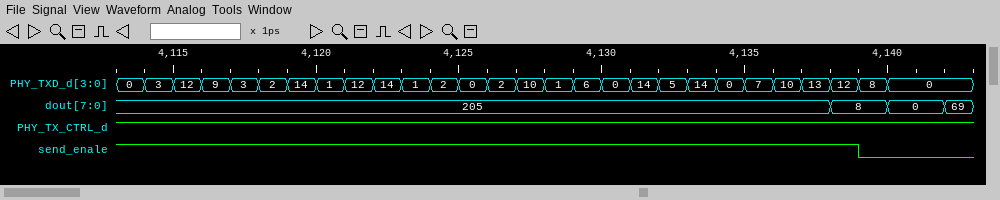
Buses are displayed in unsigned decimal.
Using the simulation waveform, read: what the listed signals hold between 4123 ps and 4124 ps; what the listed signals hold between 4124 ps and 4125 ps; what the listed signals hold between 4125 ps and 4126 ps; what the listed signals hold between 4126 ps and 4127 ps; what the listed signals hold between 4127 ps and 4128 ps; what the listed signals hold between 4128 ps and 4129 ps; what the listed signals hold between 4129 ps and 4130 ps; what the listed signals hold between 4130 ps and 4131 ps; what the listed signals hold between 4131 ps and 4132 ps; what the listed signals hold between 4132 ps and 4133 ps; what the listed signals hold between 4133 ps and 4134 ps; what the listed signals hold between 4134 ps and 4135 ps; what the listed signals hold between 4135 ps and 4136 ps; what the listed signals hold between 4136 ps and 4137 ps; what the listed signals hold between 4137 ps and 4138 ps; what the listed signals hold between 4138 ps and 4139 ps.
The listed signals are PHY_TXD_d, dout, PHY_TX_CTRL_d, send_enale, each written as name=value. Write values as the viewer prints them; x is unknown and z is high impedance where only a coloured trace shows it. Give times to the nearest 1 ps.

PHY_TXD_d=1, dout=205, PHY_TX_CTRL_d=1, send_enale=1
PHY_TXD_d=2, dout=205, PHY_TX_CTRL_d=1, send_enale=1
PHY_TXD_d=0, dout=205, PHY_TX_CTRL_d=1, send_enale=1
PHY_TXD_d=2, dout=205, PHY_TX_CTRL_d=1, send_enale=1
PHY_TXD_d=10, dout=205, PHY_TX_CTRL_d=1, send_enale=1
PHY_TXD_d=1, dout=205, PHY_TX_CTRL_d=1, send_enale=1
PHY_TXD_d=6, dout=205, PHY_TX_CTRL_d=1, send_enale=1
PHY_TXD_d=0, dout=205, PHY_TX_CTRL_d=1, send_enale=1
PHY_TXD_d=14, dout=205, PHY_TX_CTRL_d=1, send_enale=1
PHY_TXD_d=5, dout=205, PHY_TX_CTRL_d=1, send_enale=1
PHY_TXD_d=14, dout=205, PHY_TX_CTRL_d=1, send_enale=1
PHY_TXD_d=0, dout=205, PHY_TX_CTRL_d=1, send_enale=1
PHY_TXD_d=7, dout=205, PHY_TX_CTRL_d=1, send_enale=1
PHY_TXD_d=10, dout=205, PHY_TX_CTRL_d=1, send_enale=1
PHY_TXD_d=13, dout=205, PHY_TX_CTRL_d=1, send_enale=1
PHY_TXD_d=12, dout=8, PHY_TX_CTRL_d=1, send_enale=1
